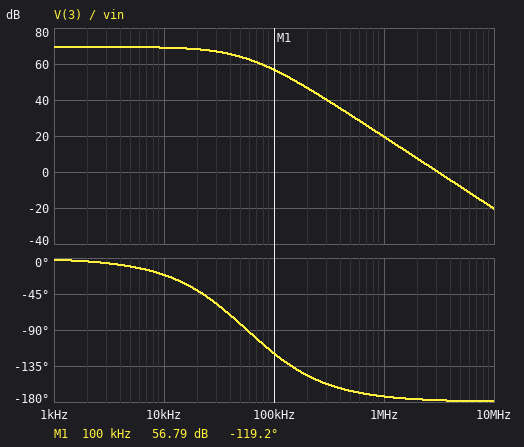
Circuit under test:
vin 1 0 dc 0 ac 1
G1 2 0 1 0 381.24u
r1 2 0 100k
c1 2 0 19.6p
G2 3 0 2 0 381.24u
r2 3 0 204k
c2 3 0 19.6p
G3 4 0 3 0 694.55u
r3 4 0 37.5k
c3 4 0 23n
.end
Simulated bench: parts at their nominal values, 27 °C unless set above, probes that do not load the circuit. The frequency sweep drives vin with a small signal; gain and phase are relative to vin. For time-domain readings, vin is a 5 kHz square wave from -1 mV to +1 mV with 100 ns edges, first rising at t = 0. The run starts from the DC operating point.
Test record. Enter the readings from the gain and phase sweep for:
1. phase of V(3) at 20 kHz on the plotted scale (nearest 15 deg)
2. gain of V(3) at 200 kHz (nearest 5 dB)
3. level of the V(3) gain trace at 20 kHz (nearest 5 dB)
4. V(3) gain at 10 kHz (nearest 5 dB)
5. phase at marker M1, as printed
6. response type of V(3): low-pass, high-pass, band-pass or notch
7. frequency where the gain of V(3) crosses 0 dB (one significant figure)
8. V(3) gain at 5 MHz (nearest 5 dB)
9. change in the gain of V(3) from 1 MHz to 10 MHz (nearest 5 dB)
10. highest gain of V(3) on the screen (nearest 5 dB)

-45 deg
45 dB
70 dB
70 dB
-119.2 deg
low-pass
3 MHz
-10 dB
-40 dB
70 dB
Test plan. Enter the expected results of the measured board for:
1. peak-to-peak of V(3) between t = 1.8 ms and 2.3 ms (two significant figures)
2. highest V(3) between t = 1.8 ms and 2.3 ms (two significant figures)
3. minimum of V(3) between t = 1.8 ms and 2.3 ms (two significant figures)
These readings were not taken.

5.9 V
3.0 V
-3.0 V
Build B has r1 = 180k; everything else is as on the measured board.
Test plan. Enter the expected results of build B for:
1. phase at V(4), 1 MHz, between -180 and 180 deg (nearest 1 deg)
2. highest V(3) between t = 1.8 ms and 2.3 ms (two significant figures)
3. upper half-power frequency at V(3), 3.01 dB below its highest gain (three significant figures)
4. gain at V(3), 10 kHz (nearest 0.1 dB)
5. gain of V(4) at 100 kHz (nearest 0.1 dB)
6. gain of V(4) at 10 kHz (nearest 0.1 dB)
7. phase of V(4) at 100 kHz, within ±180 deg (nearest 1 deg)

-85 deg
5.3 V
27.2 kHz
74.1 dB
31.8 dB
67.7 dB
-44 deg
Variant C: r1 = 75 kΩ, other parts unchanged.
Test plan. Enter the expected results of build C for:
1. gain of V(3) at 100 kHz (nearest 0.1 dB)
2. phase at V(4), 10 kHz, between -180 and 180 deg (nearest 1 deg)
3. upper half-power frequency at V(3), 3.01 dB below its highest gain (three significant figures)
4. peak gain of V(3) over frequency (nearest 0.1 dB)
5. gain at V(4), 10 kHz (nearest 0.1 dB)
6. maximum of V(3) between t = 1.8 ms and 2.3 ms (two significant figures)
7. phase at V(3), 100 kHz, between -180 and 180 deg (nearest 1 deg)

55.6 dB
72 deg
35.7 kHz
66.9 dB
60.3 dB
2.2 V
-111 deg
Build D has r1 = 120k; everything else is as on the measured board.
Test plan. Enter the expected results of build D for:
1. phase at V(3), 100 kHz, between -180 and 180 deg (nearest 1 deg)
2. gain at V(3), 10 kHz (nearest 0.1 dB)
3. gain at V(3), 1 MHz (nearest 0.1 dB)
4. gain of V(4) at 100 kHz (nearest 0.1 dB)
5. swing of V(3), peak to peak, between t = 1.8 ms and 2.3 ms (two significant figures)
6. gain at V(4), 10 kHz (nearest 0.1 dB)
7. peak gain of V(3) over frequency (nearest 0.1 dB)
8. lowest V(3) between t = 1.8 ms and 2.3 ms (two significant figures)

-124 deg
70.7 dB
19.6 dB
31.0 dB
7.1 V
64.3 dB
71.0 dB
-3.6 V
